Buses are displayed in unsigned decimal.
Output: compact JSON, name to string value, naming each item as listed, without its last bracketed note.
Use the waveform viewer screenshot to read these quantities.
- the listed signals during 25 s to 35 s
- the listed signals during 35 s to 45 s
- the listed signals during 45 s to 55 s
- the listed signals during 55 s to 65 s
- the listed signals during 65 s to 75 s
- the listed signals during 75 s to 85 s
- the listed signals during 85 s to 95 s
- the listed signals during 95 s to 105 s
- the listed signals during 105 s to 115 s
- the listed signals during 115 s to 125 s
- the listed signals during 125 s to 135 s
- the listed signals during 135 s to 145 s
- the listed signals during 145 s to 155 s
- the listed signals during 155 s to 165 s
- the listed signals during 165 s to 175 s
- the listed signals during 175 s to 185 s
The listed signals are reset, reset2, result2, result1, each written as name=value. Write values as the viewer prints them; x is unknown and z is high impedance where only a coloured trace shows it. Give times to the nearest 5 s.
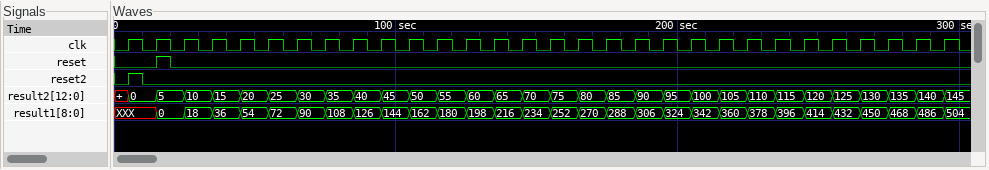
{"the listed signals during 25 s to 35 s": "reset=0, reset2=0, result2=10, result1=18", "the listed signals during 35 s to 45 s": "reset=0, reset2=0, result2=15, result1=36", "the listed signals during 45 s to 55 s": "reset=0, reset2=0, result2=20, result1=54", "the listed signals during 55 s to 65 s": "reset=0, reset2=0, result2=25, result1=72", "the listed signals during 65 s to 75 s": "reset=0, reset2=0, result2=30, result1=90", "the listed signals during 75 s to 85 s": "reset=0, reset2=0, result2=35, result1=108", "the listed signals during 85 s to 95 s": "reset=0, reset2=0, result2=40, result1=126", "the listed signals during 95 s to 105 s": "reset=0, reset2=0, result2=45, result1=144", "the listed signals during 105 s to 115 s": "reset=0, reset2=0, result2=50, result1=162", "the listed signals during 115 s to 125 s": "reset=0, reset2=0, result2=55, result1=180", "the listed signals during 125 s to 135 s": "reset=0, reset2=0, result2=60, result1=198", "the listed signals during 135 s to 145 s": "reset=0, reset2=0, result2=65, result1=216", "the listed signals during 145 s to 155 s": "reset=0, reset2=0, result2=70, result1=234", "the listed signals during 155 s to 165 s": "reset=0, reset2=0, result2=75, result1=252", "the listed signals during 165 s to 175 s": "reset=0, reset2=0, result2=80, result1=270", "the listed signals during 175 s to 185 s": "reset=0, reset2=0, result2=85, result1=288"}
